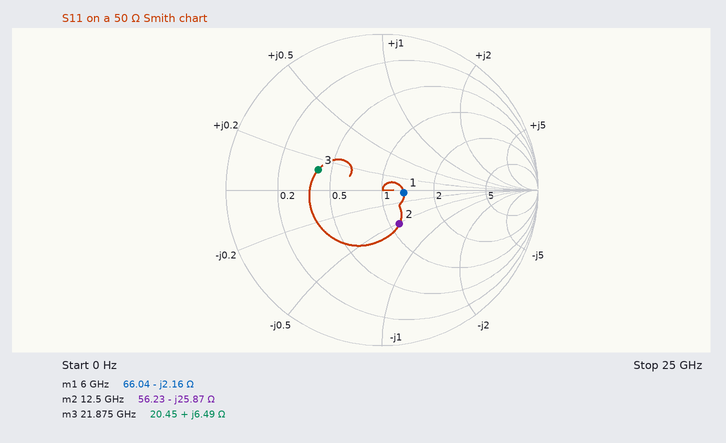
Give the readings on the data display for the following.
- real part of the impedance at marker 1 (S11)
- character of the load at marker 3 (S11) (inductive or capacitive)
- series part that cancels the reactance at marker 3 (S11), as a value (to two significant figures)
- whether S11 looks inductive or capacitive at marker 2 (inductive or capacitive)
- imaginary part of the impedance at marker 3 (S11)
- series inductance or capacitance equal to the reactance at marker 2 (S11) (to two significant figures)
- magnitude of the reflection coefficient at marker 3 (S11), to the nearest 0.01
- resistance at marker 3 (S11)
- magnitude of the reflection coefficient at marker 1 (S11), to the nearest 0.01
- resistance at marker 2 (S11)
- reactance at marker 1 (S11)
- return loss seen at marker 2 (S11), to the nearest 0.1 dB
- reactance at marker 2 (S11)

66.04 Ω
inductive
1.1 pF
capacitive
+6.49 Ω
490 fF
0.43
20.45 Ω
0.14
56.23 Ω
-2.16 Ω
12.3 dB
-25.87 Ω
